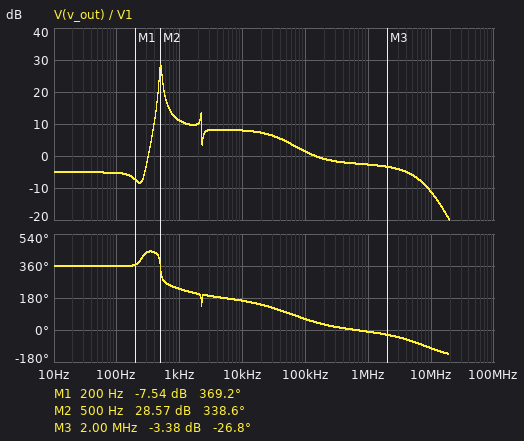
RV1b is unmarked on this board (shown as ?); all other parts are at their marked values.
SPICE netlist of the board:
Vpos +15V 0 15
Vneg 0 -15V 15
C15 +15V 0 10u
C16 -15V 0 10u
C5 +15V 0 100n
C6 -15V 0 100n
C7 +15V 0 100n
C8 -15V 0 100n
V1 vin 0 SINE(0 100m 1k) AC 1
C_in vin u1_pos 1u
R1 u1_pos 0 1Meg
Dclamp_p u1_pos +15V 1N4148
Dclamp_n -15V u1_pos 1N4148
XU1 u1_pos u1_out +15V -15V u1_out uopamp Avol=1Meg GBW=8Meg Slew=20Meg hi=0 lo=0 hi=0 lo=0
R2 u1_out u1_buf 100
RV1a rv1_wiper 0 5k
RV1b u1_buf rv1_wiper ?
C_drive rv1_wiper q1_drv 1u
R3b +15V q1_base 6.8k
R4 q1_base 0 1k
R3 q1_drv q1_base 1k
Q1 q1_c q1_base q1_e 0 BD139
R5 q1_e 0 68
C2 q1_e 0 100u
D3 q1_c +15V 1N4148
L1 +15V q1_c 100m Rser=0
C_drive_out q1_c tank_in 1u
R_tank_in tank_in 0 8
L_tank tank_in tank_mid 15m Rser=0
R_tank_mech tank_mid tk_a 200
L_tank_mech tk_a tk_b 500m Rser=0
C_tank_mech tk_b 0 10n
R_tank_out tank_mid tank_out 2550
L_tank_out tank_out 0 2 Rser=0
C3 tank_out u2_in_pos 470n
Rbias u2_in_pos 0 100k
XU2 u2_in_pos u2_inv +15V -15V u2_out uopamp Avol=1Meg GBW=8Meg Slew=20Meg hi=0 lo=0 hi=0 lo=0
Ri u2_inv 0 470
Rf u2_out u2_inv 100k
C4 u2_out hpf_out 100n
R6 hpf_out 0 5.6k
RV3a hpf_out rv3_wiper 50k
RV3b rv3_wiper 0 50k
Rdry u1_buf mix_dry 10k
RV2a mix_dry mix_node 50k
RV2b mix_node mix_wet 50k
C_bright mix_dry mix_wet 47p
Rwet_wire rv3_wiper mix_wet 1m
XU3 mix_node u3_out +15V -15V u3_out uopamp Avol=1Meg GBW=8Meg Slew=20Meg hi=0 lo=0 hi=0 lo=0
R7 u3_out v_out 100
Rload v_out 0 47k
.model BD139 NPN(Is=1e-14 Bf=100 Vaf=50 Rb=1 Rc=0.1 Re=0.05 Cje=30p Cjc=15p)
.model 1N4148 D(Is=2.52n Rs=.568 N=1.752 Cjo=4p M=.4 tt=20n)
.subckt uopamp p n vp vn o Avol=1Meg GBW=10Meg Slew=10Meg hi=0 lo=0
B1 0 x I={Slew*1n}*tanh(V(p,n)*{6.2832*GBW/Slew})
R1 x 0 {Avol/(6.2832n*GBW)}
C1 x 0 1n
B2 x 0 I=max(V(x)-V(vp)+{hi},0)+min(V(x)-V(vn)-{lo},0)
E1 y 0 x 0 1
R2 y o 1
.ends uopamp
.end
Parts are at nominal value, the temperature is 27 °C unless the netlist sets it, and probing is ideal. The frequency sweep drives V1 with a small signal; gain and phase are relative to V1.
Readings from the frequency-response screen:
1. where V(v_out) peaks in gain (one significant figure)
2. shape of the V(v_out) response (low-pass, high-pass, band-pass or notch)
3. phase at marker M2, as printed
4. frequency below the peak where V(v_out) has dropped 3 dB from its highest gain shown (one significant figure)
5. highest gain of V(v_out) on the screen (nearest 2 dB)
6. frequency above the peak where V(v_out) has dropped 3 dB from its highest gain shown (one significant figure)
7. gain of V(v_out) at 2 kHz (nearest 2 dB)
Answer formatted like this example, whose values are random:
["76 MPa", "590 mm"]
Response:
["500 Hz", "band-pass", "338.6 deg", "500 Hz", "28 dB", "500 Hz", "10 dB"]
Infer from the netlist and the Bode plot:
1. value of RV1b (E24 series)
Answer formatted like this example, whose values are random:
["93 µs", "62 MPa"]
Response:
["8.2 kΩ"]
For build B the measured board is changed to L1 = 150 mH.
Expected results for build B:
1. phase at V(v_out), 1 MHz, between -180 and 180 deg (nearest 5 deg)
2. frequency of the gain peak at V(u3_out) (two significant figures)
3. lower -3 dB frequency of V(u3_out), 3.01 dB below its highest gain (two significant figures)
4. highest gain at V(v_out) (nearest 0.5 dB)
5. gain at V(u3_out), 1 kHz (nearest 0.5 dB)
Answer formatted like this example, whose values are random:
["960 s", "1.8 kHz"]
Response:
["-10 deg", "400 Hz", "390 Hz", "27.0 dB", "10.0 dB"]
